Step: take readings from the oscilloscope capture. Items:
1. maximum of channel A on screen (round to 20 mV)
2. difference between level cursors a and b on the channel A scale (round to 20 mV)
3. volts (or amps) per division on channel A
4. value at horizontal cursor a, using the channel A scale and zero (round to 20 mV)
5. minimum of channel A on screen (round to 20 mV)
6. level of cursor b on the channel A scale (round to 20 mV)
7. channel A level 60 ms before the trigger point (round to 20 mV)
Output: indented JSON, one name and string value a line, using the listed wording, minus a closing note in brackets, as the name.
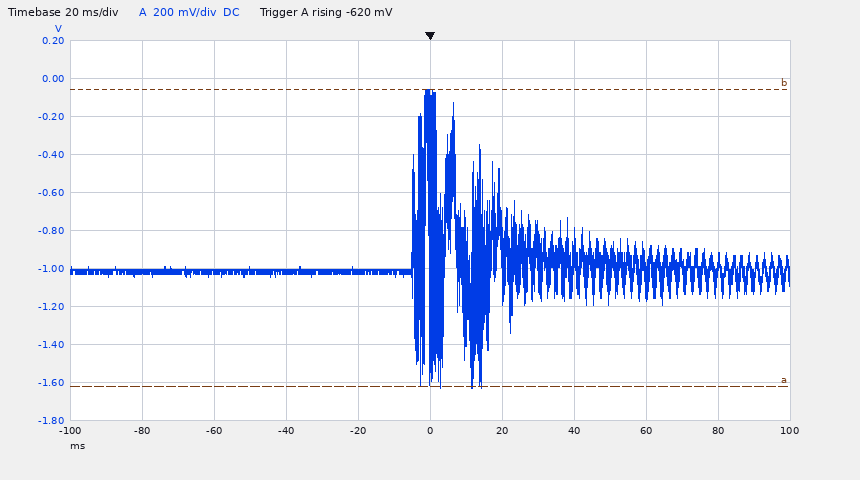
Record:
{
  "maximum of channel A on screen": "-60 mV",
  "difference between level cursors a and b on the channel A scale": "1.56 V",
  "volts (or amps) per division on channel A": "200 mV",
  "value at horizontal cursor a, using the channel A scale and zero": "-1.62 V",
  "minimum of channel A on screen": "-1.62 V",
  "level of cursor b on the channel A scale": "-60 mV",
  "channel A level 60 ms before the trigger point": "-1.02 V"
}
